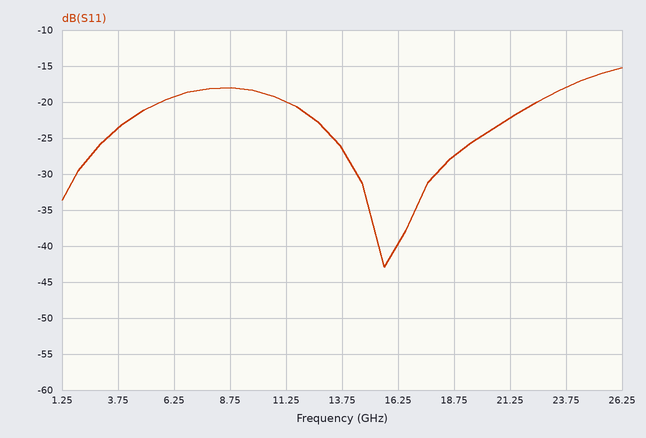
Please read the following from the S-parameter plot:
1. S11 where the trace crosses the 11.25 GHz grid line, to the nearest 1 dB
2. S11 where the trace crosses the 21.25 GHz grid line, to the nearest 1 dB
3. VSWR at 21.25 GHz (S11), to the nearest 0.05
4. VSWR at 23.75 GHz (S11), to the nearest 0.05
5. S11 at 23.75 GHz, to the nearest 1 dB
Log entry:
-20 dB
-22 dB
1.15
1.30
-18 dB
